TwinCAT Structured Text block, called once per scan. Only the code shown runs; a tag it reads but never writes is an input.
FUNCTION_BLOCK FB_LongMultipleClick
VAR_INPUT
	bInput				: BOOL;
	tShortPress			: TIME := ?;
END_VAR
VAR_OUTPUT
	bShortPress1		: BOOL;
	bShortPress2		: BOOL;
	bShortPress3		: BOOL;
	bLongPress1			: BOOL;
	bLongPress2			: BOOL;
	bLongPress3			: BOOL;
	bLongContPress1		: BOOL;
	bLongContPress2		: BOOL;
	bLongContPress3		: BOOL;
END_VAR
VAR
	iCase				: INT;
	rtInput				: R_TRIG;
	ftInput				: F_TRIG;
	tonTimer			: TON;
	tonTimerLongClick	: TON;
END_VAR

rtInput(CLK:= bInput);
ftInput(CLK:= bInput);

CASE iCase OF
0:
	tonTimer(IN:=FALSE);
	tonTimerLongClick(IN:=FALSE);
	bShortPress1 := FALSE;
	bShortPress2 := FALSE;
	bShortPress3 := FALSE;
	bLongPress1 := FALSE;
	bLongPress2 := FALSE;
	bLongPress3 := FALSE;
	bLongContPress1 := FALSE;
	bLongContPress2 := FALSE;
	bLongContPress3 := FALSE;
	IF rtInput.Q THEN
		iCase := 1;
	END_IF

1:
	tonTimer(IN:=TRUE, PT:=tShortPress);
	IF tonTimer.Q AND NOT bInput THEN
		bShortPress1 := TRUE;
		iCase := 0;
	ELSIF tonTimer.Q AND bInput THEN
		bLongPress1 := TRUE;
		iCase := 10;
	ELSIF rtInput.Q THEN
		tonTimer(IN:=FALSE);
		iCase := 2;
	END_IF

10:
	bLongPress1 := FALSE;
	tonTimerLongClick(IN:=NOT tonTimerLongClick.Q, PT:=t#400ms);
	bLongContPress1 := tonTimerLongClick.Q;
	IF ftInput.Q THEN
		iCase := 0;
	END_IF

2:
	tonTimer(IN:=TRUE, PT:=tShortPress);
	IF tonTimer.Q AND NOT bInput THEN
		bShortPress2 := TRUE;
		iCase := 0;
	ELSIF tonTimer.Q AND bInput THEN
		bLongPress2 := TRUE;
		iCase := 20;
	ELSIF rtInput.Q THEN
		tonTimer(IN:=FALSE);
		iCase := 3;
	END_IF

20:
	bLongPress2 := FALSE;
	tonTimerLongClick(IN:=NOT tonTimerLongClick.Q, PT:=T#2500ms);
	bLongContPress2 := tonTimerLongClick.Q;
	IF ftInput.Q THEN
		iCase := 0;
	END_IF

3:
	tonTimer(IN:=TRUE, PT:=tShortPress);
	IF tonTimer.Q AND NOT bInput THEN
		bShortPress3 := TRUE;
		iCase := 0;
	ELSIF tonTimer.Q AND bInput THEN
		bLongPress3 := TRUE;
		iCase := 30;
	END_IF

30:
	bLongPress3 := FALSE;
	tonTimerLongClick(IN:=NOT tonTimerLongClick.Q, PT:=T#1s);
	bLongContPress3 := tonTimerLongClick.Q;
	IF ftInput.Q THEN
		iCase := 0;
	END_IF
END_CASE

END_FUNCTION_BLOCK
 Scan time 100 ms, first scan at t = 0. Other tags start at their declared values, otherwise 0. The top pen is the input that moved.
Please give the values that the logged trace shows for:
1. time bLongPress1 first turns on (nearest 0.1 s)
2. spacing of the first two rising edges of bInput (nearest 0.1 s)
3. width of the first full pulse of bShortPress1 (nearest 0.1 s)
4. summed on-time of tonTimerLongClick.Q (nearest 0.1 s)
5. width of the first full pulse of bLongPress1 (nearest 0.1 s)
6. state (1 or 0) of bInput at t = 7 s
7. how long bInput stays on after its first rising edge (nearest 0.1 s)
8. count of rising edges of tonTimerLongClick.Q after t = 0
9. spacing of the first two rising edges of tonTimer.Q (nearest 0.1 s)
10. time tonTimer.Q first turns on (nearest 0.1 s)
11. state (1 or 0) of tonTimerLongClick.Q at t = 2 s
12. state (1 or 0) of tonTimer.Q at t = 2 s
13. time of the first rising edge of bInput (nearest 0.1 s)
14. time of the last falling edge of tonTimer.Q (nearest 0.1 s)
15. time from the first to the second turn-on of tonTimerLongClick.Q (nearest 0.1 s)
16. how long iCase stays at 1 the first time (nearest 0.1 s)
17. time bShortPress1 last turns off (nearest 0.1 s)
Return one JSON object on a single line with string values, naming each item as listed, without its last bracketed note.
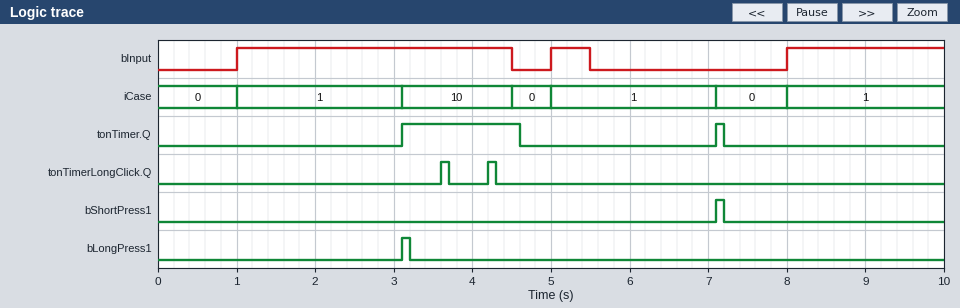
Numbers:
{"time bLongPress1 first turns on": "3.1 s", "spacing of the first two rising edges of bInput": "4.0 s", "width of the first full pulse of bShortPress1": "0.1 s", "summed on-time of tonTimerLongClick.Q": "0.2 s", "width of the first full pulse of bLongPress1": "0.1 s", "state (1 or 0) of bInput at t = 7 s": "0", "how long bInput stays on after its first rising edge": "3.5 s", "count of rising edges of tonTimerLongClick.Q after t = 0": "2", "spacing of the first two rising edges of tonTimer.Q": "4.0 s", "time tonTimer.Q first turns on": "3.1 s", "state (1 or 0) of tonTimerLongClick.Q at t = 2 s": "0", "state (1 or 0) of tonTimer.Q at t = 2 s": "0", "time of the first rising edge of bInput": "1.0 s", "time of the last falling edge of tonTimer.Q": "7.2 s", "time from the first to the second turn-on of tonTimerLongClick.Q": "0.6 s", "how long iCase stays at 1 the first time": "2.1 s", "time bShortPress1 last turns off": "7.2 s"}
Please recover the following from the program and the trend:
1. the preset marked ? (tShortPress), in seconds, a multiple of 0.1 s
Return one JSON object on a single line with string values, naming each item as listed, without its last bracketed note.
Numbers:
{"the preset marked ? (tShortPress), in seconds, a multiple of 0.1 s": "2.0 s"}
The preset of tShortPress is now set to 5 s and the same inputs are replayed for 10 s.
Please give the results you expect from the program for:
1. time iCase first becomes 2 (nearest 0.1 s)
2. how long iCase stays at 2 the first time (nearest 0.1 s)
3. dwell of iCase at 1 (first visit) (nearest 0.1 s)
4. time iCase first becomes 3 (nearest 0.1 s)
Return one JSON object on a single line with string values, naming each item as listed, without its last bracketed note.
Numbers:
{"time iCase first becomes 2": "5.0 s", "how long iCase stays at 2 the first time": "3.0 s", "dwell of iCase at 1 (first visit)": "4.0 s", "time iCase first becomes 3": "8.0 s"}
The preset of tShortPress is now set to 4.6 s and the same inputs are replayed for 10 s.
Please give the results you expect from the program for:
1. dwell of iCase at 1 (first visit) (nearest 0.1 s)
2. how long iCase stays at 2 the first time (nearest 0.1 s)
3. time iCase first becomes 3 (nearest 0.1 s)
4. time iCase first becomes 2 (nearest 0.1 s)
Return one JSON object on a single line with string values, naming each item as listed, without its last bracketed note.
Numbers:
{"dwell of iCase at 1 (first visit)": "4.0 s", "how long iCase stays at 2 the first time": "3.0 s", "time iCase first becomes 3": "8.0 s", "time iCase first becomes 2": "5.0 s"}
